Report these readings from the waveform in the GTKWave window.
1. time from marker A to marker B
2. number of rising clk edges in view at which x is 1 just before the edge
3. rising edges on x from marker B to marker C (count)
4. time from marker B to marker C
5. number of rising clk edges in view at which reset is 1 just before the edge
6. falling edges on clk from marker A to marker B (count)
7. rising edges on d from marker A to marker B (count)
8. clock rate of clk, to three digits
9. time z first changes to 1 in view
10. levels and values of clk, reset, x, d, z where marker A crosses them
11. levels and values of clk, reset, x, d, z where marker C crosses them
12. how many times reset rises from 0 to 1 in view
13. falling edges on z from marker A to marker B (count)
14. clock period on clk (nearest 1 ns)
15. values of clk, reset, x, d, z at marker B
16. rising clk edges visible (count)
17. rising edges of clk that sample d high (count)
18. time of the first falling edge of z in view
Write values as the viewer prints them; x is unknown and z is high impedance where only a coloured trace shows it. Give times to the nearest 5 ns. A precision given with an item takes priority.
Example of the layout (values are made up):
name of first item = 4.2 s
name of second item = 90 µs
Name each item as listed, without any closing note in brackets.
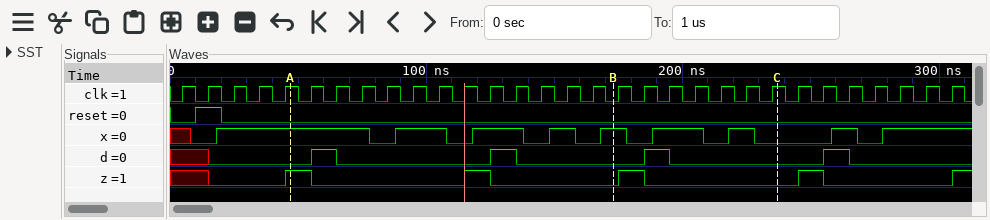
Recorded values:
time from marker A to marker B = 125 ns
number of rising clk edges in view at which x is 1 just before the edge = 19
rising edges on x from marker B to marker C = 2
time from marker B to marker C = 65 ns
number of rising clk edges in view at which reset is 1 just before the edge = 1
falling edges on clk from marker A to marker B = 13
rising edges on d from marker A to marker B = 2
clock rate of clk, to three digits = 100 MHz
time z first changes to 1 in view = 45 ns
levels and values of clk, reset, x, d, z where marker A crosses them = clk=1, reset=0, x=1, d=0, z=1
levels and values of clk, reset, x, d, z where marker C crosses them = clk=1, reset=0, x=0, d=0, z=0
how many times reset rises from 0 to 1 in view = 1
falling edges on z from marker A to marker B = 2
clock period on clk = 10 ns
values of clk, reset, x, d, z at marker B = clk=0, reset=0, x=1, d=0, z=0
rising clk edges visible = 31
rising edges of clk that sample d high = 4
time of the first falling edge of z in view = 55 ns
